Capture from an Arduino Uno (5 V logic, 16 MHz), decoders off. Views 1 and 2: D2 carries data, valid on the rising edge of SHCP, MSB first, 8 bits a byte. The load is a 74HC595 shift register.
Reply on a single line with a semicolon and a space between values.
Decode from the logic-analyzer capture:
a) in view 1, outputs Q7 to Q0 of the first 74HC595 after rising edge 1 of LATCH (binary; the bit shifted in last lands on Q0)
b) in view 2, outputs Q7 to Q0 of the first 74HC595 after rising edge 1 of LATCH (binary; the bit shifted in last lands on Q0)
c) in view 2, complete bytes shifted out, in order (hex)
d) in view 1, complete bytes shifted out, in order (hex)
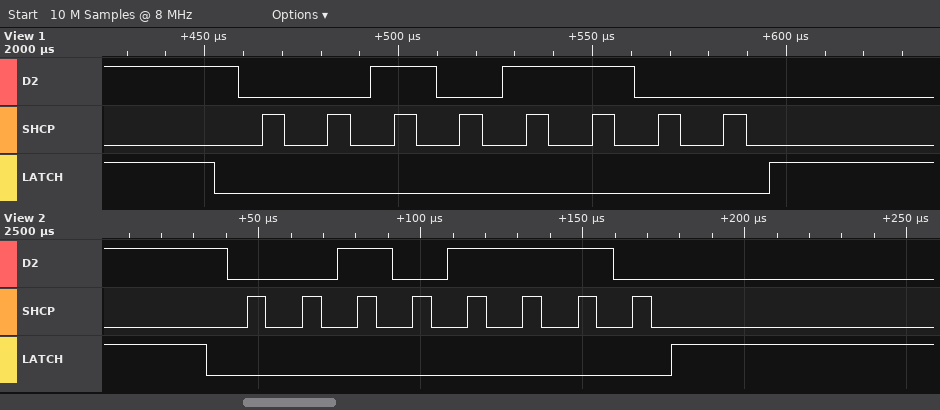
00101100; 00101110; 2E; 2C
